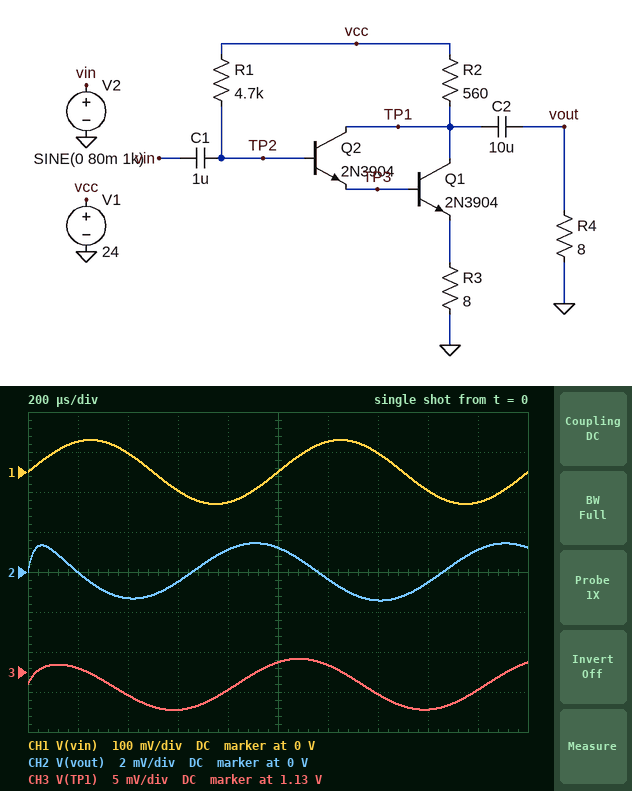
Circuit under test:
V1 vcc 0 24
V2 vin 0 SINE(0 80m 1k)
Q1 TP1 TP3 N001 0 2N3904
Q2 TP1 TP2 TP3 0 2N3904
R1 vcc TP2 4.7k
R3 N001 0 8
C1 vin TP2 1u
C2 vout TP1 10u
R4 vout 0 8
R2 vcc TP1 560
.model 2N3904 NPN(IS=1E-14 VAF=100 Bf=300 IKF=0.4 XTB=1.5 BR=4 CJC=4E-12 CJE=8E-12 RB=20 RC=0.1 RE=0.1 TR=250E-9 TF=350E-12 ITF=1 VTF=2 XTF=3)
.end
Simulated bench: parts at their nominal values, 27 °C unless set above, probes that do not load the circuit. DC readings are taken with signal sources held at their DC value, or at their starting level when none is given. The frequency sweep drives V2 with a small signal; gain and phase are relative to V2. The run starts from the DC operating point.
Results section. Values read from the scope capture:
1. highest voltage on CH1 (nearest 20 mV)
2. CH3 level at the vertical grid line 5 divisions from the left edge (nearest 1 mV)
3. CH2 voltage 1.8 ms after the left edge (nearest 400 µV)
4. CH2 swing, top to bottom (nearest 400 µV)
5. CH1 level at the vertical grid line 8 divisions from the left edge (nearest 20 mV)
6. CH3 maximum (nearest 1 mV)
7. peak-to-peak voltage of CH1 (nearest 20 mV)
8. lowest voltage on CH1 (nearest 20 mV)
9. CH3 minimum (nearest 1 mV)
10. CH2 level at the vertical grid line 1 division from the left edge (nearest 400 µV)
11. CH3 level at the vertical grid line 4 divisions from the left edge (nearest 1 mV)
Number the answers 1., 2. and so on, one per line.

1. 80 mV
2. 1.131 V
3. 1.2 mV
4. 2.8 mV
5. -40 mV
6. 1.132 V
7. 160 mV
8. -80 mV
9. 1.125 V
10. 0 V
11. 1.128 V
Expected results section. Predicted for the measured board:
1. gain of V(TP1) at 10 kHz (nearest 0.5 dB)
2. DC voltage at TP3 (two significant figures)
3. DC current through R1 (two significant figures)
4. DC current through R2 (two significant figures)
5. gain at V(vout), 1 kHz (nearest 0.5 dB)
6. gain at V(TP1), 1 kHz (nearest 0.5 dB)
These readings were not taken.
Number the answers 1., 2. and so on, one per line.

1. -18.5 dB
2. 1.1 V
3. 4.7 mA
4. 41 mA
5. -35.0 dB
6. -28.0 dB
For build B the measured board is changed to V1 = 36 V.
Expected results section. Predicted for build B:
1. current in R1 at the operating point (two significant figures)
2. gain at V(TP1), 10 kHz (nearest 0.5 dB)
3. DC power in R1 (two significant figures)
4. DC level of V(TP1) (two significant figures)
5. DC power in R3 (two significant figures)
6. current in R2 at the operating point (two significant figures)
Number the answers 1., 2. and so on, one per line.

1. 7.2 mA
2. -18.0 dB
3. 240 mW
4. 1.3 V
5. 38 mW
6. 62 mA
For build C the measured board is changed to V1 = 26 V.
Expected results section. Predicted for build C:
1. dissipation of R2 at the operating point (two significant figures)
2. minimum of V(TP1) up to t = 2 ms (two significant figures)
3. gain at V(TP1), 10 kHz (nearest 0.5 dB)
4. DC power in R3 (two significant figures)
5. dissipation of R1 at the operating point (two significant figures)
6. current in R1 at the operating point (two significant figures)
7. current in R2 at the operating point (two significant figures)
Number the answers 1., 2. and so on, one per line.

1. 1.1 W
2. 1.2 V
3. -18.0 dB
4. 20 mW
5. 120 mW
6. 5.1 mA
7. 44 mA
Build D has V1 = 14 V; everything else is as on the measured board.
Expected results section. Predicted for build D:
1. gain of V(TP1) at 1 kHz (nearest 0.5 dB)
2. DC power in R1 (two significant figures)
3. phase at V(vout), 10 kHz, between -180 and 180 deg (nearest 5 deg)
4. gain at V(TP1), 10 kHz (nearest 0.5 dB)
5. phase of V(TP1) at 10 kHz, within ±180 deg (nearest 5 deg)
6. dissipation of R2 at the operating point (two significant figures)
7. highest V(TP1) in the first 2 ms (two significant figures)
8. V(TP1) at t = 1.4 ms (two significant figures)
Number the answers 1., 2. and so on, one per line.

1. -28.0 dB
2. 32 mW
3. 30 deg
4. -19.0 dB
5. 20 deg
6. 300 mW
7. 960 mV
8. 950 mV
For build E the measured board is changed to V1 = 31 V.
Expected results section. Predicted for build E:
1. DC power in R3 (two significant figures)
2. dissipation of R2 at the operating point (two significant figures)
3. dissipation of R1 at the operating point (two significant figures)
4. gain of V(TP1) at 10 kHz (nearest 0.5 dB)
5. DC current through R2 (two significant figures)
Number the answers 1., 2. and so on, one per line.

1. 28 mW
2. 1.6 W
3. 180 mW
4. -18.0 dB
5. 53 mA
